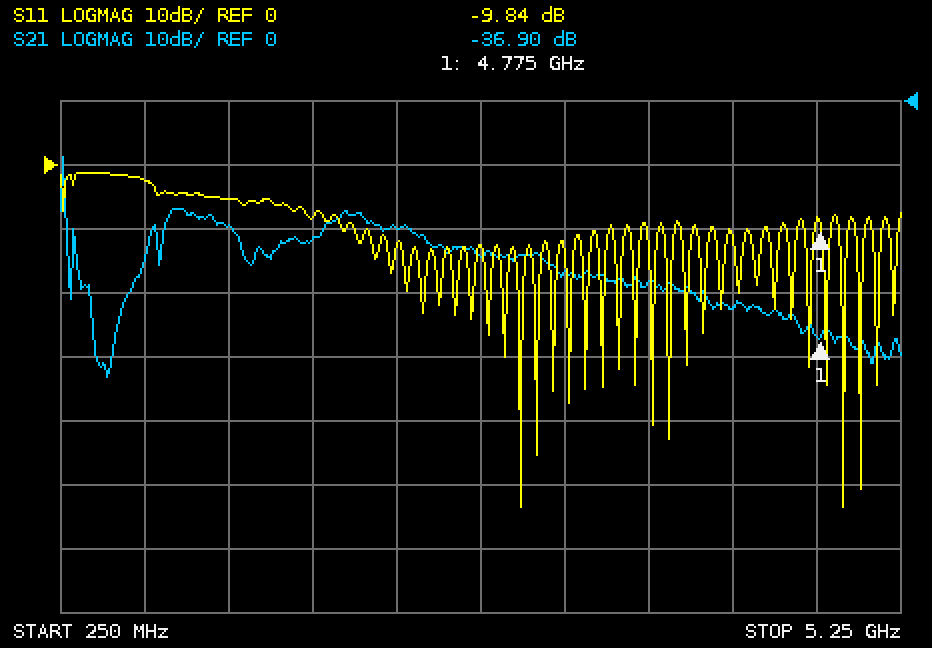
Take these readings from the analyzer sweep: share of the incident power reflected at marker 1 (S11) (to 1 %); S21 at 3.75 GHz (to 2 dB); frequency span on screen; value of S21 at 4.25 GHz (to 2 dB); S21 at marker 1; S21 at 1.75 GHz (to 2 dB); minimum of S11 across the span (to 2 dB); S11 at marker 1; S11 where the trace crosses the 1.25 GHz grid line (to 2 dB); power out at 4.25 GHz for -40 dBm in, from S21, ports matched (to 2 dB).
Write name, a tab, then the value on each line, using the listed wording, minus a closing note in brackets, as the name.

share of the incident power reflected at marker 1 (S11)	10 %
S21 at 3.75 GHz	-28 dB
frequency span on screen	5 GHz
value of S21 at 4.25 GHz	-32 dB
S21 at marker 1	-36.90 dB
S21 at 1.75 GHz	-22 dB
minimum of S11 across the span	-54 dB
S11 at marker 1	-9.84 dB
S11 where the trace crosses the 1.25 GHz grid line	-6 dB
power out at 4.25 GHz for -40 dBm in, from S21, ports matched	-72 dBm
